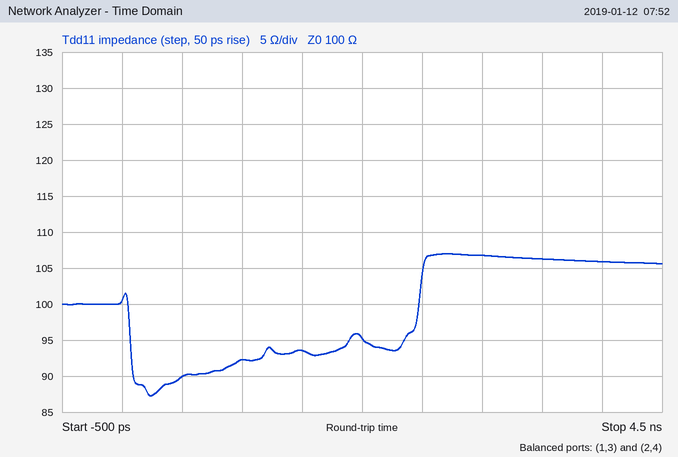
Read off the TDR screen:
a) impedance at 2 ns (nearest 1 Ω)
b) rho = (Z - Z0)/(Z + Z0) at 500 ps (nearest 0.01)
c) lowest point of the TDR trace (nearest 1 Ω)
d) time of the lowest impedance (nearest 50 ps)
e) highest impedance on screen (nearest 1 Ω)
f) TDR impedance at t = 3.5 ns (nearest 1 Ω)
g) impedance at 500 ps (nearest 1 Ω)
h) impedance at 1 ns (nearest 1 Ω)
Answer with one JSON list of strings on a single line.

["95 Ω", "-0.05", "87 Ω", "250 ps", "107 Ω", "106 Ω", "90 Ω", "92 Ω"]
